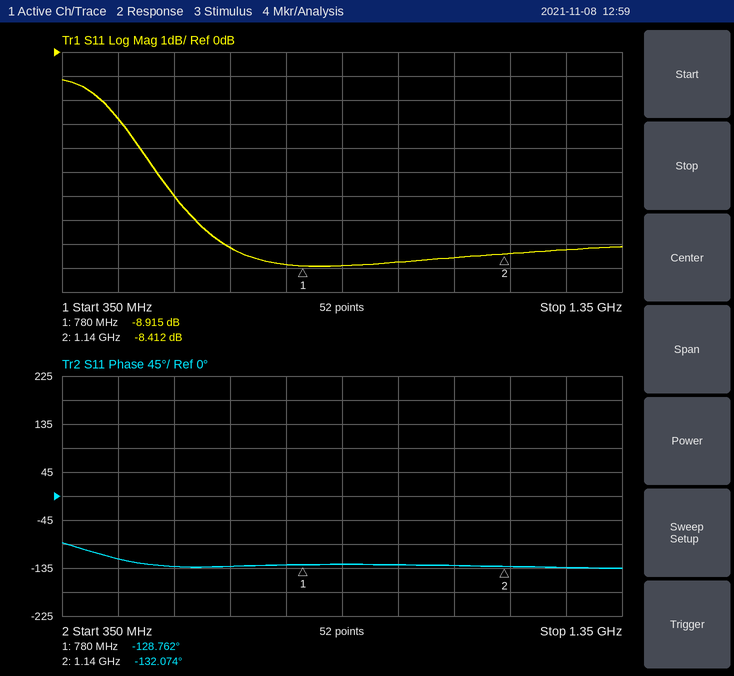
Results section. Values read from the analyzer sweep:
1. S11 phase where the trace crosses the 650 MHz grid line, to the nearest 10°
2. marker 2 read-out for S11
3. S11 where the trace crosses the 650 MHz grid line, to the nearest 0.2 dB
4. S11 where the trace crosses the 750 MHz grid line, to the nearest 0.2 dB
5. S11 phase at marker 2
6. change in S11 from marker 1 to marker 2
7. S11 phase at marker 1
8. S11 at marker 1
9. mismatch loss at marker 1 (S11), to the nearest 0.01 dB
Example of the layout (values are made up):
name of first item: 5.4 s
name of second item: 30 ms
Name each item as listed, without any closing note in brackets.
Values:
S11 phase where the trace crosses the 650 MHz grid line, to the nearest 10°: -130°
marker 2 read-out for S11: -8.412 dB
S11 where the trace crosses the 650 MHz grid line, to the nearest 0.2 dB: -8.2 dB
S11 where the trace crosses the 750 MHz grid line, to the nearest 0.2 dB: -8.8 dB
S11 phase at marker 2: -132.074°
change in S11 from marker 1 to marker 2: 0.503 dB
S11 phase at marker 1: -128.762°
S11 at marker 1: -8.915 dB
mismatch loss at marker 1 (S11), to the nearest 0.01 dB: 0.60 dB
